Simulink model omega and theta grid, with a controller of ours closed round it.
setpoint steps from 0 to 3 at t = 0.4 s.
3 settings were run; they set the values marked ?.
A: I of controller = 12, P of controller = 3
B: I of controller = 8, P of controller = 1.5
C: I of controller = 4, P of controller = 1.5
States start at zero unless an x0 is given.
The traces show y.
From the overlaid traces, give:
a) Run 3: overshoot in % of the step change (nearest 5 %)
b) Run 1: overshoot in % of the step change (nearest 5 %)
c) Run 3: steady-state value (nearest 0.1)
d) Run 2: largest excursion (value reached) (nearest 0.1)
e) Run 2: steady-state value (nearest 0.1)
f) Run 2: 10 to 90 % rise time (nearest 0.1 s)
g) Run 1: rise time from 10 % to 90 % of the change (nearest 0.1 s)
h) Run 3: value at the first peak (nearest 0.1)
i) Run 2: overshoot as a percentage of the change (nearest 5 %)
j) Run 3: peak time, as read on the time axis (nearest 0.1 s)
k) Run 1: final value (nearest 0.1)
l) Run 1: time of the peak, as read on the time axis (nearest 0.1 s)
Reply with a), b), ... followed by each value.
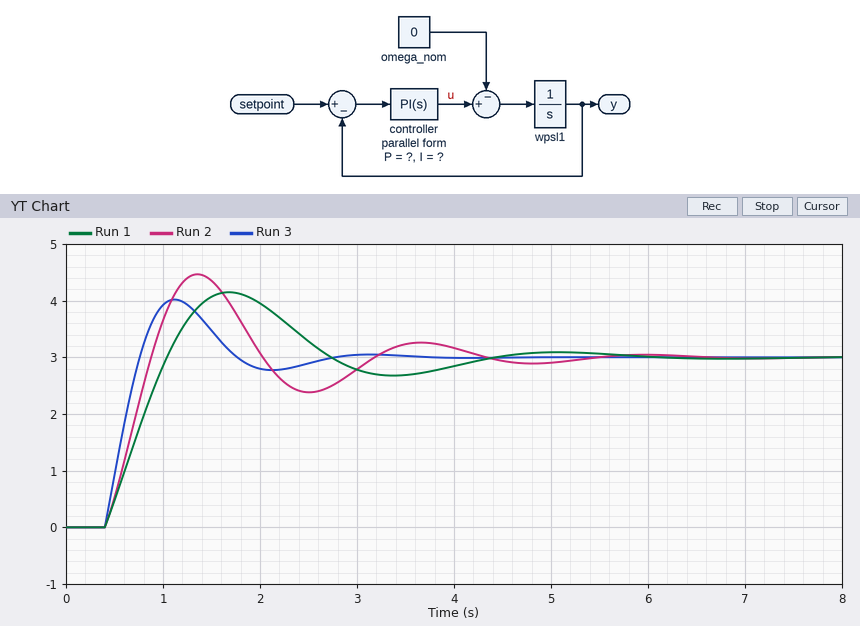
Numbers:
a) 35 %
b) 40 %
c) 3.0
d) 4.5
e) 3.0
f) 0.4 s
g) 0.5 s
h) 4.0
i) 50 %
j) 1.1 s
k) 3.0
l) 1.7 s
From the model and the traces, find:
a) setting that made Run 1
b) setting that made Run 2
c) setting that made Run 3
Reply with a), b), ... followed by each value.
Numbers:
a) C
b) B
c) A
